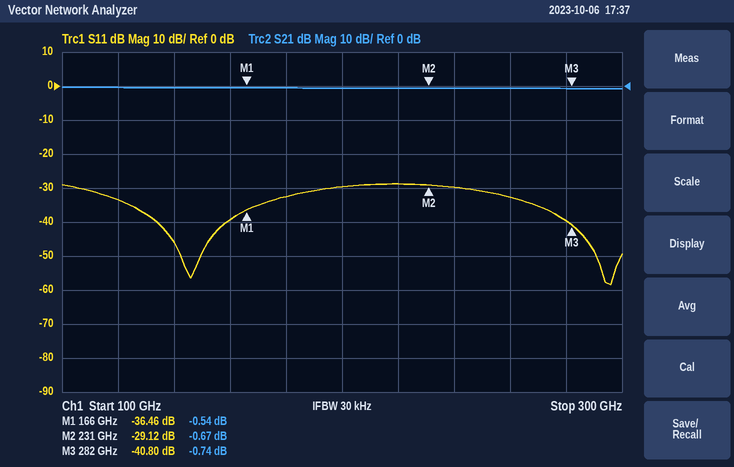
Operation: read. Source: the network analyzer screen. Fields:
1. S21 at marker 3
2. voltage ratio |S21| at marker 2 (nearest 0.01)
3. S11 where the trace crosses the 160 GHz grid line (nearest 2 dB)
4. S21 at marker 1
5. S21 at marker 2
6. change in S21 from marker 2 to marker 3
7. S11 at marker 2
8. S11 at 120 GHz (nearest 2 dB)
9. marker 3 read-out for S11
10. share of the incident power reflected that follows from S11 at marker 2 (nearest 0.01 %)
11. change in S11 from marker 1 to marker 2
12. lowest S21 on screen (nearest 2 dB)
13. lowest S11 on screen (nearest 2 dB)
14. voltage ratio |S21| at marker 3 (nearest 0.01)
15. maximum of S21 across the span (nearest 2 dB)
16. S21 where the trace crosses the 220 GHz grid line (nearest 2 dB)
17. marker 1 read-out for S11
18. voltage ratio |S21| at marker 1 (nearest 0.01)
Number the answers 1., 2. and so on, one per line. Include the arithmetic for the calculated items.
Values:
1. -0.74 dB
2. 10^(-0.67/20) ≈ 0.93
3. -40 dB
4. -0.54 dB
5. -0.67 dB
6. -0.74 − (-0.67) = -0.07 dB
7. -29.12 dB
8. -34 dB
9. -40.80 dB
10. 10^(-29.12/10) ≈ 0.12 %
11. -29.12 − (-36.46) = 7.34 dB
12. 0 dB
13. -58 dB
14. 10^(-0.74/20) ≈ 0.92
15. 0 dB
16. 0 dB
17. -36.46 dB
18. 10^(-0.54/20) ≈ 0.94
